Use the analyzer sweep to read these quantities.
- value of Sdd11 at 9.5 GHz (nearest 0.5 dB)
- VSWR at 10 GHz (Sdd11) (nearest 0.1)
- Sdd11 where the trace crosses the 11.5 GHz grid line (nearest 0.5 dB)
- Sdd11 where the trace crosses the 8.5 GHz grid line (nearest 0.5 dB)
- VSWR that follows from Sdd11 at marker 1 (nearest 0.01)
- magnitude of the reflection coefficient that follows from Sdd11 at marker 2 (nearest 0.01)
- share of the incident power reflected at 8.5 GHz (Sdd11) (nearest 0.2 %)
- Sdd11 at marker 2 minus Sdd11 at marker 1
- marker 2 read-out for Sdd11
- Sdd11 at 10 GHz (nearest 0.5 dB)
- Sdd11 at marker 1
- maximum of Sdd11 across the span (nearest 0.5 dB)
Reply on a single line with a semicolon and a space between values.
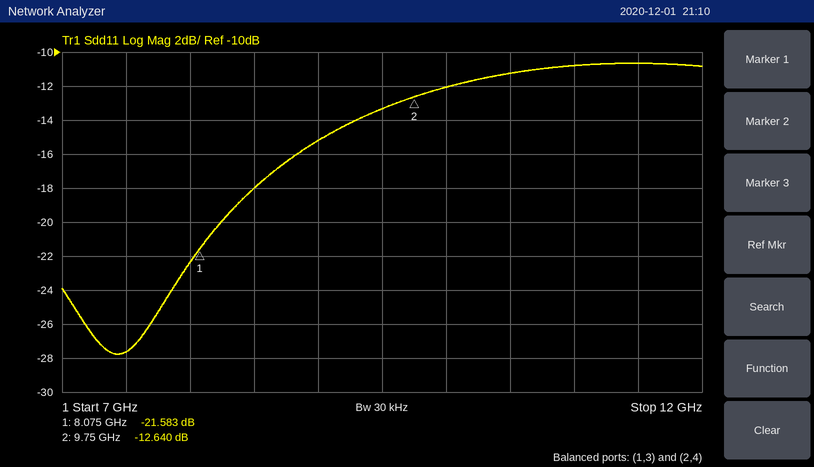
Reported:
-13.5 dB; 1.7; -10.5 dB; -18.0 dB; 1.18; 0.23; 1.6 %; 8.943 dB; -12.640 dB; -12.0 dB; -21.583 dB; -10.5 dB
